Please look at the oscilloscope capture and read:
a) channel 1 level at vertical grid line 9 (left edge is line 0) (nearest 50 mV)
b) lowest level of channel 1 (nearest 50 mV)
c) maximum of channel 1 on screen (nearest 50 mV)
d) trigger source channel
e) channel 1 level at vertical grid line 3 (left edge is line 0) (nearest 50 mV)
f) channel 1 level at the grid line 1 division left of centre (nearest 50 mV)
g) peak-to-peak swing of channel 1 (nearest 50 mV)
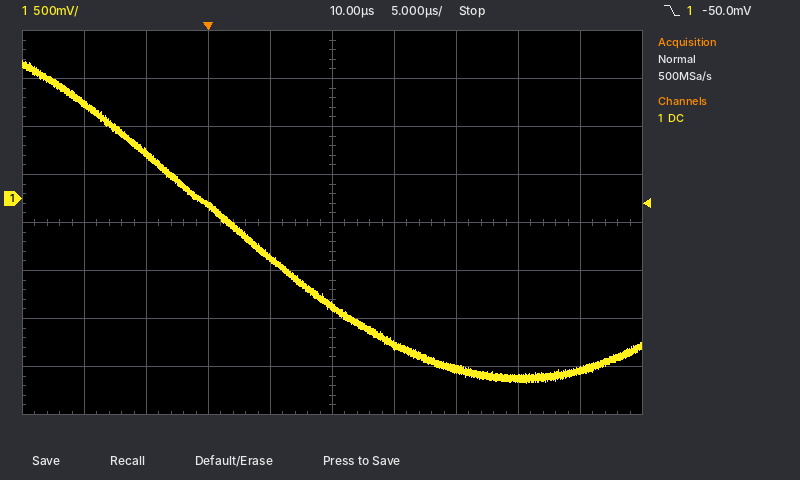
-1.80 V
-1.90 V
1.45 V
channel 1
-50 mV
-600 mV
3.35 V
